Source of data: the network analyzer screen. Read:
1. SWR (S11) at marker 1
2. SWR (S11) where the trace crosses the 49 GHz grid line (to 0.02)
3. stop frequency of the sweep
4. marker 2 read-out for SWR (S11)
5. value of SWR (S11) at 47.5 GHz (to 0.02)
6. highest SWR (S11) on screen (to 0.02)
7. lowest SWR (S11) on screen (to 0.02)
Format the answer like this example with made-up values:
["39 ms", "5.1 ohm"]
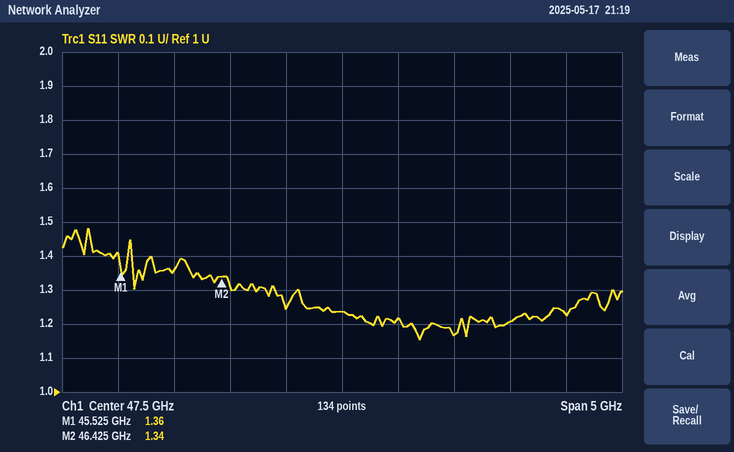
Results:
["1.36", "1.20", "50 GHz", "1.34", "1.24", "1.48", "1.16"]
